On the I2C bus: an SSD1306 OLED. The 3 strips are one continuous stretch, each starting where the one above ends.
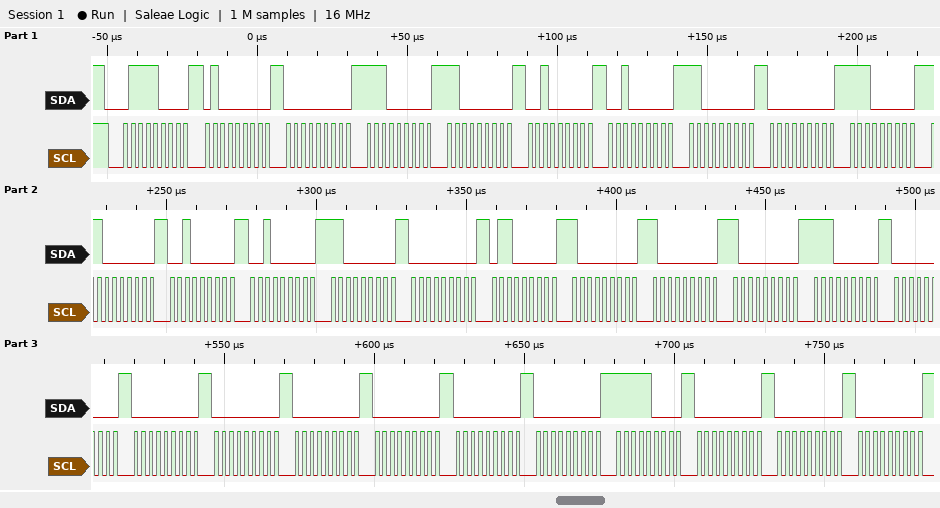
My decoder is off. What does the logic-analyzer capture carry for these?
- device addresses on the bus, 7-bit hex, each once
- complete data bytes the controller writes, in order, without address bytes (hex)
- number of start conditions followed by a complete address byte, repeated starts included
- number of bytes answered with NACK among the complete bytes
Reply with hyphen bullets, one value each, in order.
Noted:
- 0x3C
- 40 00 E0 C0 20 20 C0 00 E0 C0 20 20 C0 00 60 80 80 80 E0 00 00 00 00 00 00 00 F8 00 00 00
- 1
- 0
